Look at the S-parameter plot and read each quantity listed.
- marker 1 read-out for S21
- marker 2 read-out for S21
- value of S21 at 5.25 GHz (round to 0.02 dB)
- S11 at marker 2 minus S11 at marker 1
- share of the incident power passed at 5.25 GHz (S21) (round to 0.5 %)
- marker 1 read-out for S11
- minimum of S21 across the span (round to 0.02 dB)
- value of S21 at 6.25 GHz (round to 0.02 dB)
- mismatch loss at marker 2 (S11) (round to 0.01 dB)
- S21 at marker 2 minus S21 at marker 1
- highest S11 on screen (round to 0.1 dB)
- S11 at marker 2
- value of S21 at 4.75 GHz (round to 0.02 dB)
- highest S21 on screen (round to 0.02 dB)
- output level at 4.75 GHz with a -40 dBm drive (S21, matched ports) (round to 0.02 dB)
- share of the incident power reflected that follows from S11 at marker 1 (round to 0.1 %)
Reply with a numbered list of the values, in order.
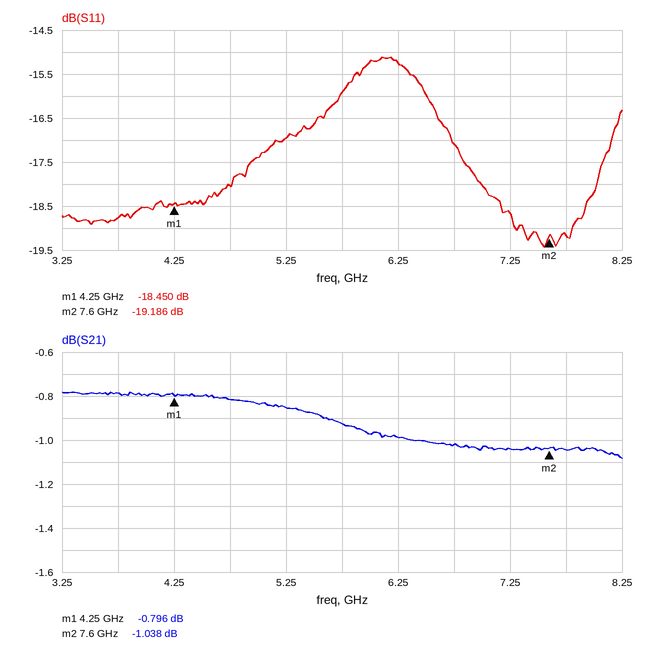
1. -0.796 dB
2. -1.038 dB
3. -0.86 dB
4. -0.736 dB
5. 82.0 %
6. -18.450 dB
7. -1.08 dB
8. -0.98 dB
9. 0.05 dB
10. -0.242 dB
11. -15.1 dB
12. -19.186 dB
13. -0.82 dB
14. -0.78 dB
15. -40.82 dBm
16. 1.4 %
